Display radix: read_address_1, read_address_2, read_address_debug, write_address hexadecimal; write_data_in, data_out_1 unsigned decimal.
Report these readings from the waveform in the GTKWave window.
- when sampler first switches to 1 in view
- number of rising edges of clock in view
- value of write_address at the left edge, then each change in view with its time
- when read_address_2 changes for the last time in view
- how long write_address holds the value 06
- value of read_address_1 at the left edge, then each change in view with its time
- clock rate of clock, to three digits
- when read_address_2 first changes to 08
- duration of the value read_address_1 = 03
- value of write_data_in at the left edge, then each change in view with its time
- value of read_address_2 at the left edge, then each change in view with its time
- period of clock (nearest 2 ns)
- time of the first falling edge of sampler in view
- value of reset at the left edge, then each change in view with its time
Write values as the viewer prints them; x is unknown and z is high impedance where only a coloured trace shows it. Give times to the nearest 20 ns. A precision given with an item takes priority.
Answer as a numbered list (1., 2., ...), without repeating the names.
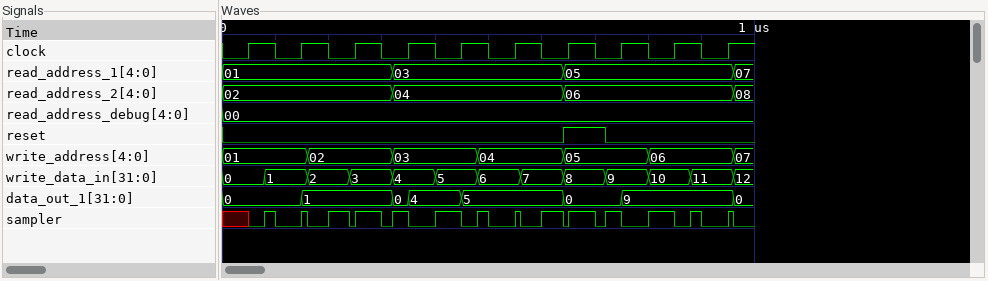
1. 80 ns
2. 10
3. 01, 02 at 160 ns, 03 at 320 ns, 04 at 480 ns, 05 at 640 ns, 06 at 800 ns, 07 at 960 ns
4. 960 ns
5. 160 ns
6. 01, 03 at 320 ns, 05 at 640 ns, 07 at 960 ns
7. 10.0 MHz
8. 960 ns
9. 320 ns
10. 0, 1 at 80 ns, 2 at 160 ns, 3 at 240 ns, 4 at 320 ns, 5 at 400 ns, 6 at 480 ns, 7 at 560 ns, 8 at 640 ns, 9 at 720 ns, 10 at 800 ns, 11 at 880 ns, 12 at 960 ns
11. 02, 04 at 320 ns, 06 at 640 ns, 08 at 960 ns
12. 100 ns
13. 100 ns
14. 0, 1 at 640 ns, 0 at 720 ns
